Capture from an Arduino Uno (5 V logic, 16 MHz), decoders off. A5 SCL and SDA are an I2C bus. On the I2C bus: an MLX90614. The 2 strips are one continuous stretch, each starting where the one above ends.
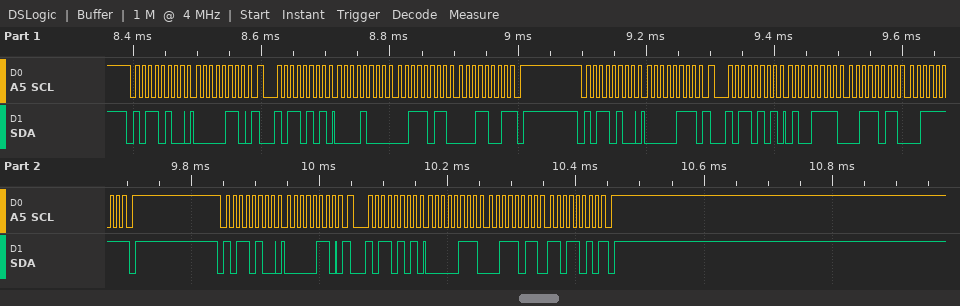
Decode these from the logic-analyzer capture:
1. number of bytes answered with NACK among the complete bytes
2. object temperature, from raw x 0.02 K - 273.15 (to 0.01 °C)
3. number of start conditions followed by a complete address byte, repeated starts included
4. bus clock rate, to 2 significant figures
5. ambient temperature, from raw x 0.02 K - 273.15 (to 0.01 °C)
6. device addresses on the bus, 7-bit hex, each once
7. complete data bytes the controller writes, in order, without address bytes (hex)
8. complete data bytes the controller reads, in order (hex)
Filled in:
3
30.51 °C
6
100 kHz
29.09 °C
0x5A
06 07 06
08 3B 19 4F 3B 3F 07 3B DA
